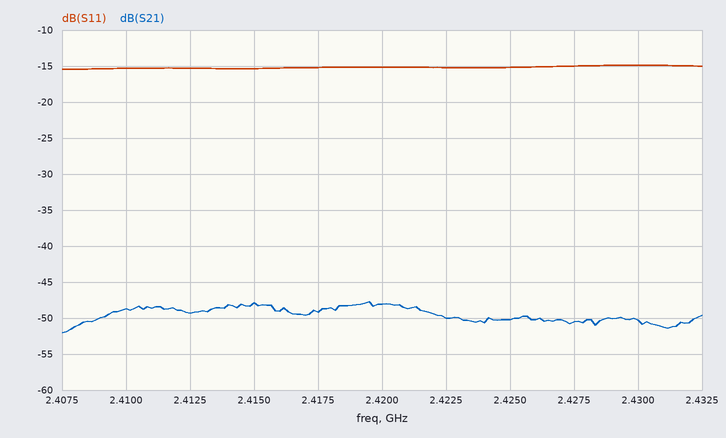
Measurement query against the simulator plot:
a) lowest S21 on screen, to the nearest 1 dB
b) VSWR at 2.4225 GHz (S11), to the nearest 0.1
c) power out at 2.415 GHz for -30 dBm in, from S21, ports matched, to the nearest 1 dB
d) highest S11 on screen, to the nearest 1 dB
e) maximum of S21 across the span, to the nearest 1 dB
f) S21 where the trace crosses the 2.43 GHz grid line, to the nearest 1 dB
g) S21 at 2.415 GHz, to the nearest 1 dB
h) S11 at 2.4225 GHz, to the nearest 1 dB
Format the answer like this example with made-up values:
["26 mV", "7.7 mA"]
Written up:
["-52 dB", "1.4", "-78 dBm", "-15 dB", "-48 dB", "-50 dB", "-48 dB", "-15 dB"]
